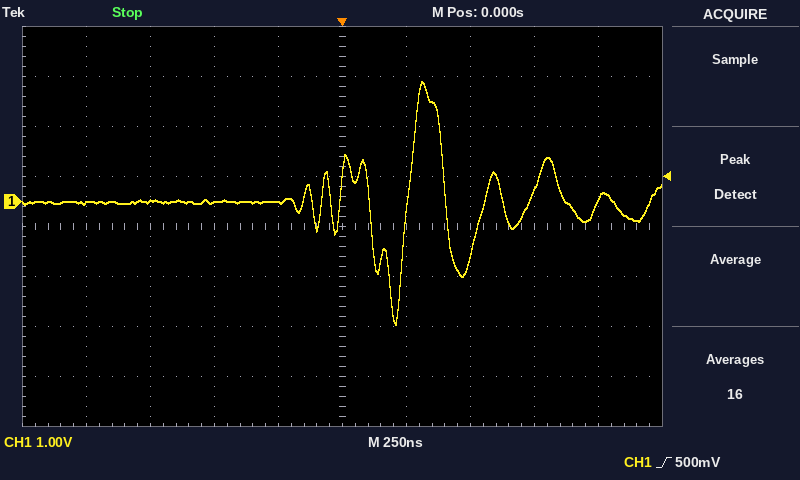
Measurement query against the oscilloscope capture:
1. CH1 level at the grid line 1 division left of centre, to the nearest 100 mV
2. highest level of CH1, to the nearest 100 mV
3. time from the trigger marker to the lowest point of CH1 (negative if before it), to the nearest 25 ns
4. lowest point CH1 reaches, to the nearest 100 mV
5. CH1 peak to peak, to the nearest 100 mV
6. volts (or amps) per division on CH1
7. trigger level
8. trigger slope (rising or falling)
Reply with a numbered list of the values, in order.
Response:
1. 0.0 V
2. 2.4 V
3. +200 ns
4. -2.5 V
5. 4.9 V
6. 1 V
7. 500 mV
8. rising
